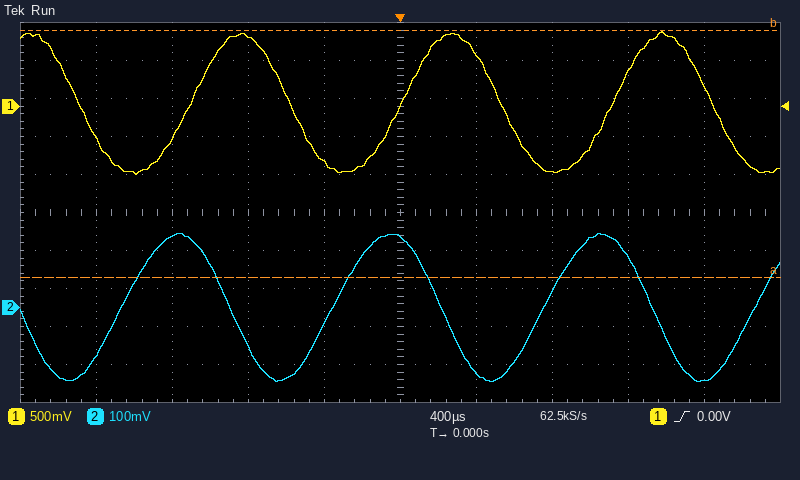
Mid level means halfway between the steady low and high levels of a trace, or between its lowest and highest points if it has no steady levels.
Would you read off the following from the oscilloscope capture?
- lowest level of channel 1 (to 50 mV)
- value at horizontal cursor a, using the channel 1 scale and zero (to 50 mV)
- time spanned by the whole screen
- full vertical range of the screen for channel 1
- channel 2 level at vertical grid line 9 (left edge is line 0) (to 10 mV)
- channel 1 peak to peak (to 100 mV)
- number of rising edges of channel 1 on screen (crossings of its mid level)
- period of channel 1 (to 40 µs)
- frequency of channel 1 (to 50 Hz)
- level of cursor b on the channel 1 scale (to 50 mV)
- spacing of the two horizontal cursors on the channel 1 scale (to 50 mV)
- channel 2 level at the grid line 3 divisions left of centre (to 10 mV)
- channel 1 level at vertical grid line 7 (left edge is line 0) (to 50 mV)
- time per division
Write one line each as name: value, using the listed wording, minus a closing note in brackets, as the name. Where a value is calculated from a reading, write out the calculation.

lowest level of channel 1: -900 mV
value at horizontal cursor a, using the channel 1 scale and zero: -2.25 V
time spanned by the whole screen: 4 ms
full vertical range of the screen for channel 1: 5 V
channel 2 level at vertical grid line 9 (left edge is line 0): -190 mV
channel 1 peak to peak: 1.90 V
number of rising edges of channel 1 on screen: 3
period of channel 1: 1.12 ms
frequency of channel 1: 1 / 1.12 ms ≈ 893 Hz, so 900 Hz to the nearest 50 Hz
level of cursor b on the channel 1 scale: 1.00 V
spacing of the two horizontal cursors on the channel 1 scale: 3.25 V
channel 2 level at the grid line 3 divisions left of centre: 190 mV
channel 1 level at vertical grid line 7 (left edge is line 0): -850 mV
time per division: 400 µs
